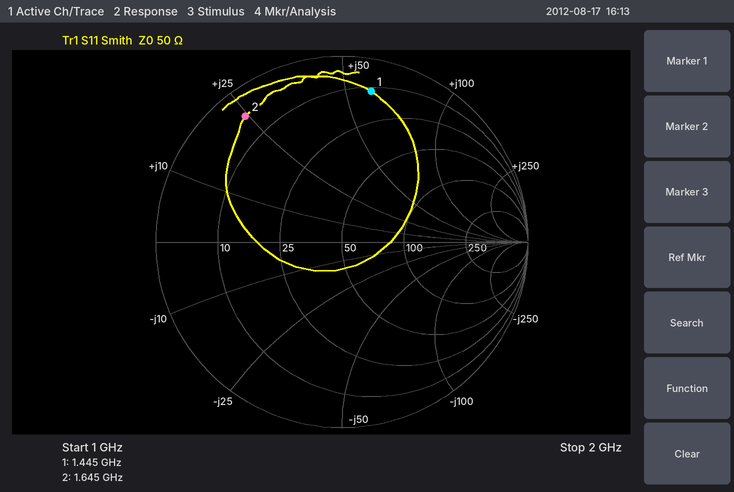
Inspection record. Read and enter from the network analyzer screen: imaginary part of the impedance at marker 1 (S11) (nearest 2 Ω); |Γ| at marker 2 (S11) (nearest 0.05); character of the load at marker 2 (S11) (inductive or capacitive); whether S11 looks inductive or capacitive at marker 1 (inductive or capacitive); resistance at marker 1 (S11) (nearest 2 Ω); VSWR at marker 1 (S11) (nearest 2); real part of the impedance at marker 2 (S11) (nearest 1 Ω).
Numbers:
+60 Ω
0.85
inductive
inductive
12 Ω
10
5 Ω
